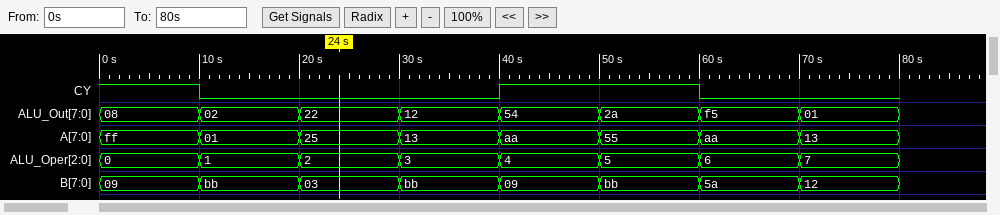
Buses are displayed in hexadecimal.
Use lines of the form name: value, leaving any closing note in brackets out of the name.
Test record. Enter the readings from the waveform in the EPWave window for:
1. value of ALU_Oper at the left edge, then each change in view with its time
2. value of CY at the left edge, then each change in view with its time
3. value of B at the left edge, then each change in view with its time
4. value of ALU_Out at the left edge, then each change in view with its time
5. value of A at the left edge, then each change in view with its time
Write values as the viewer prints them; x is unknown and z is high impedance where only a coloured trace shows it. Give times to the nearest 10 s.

value of ALU_Oper at the left edge, then each change in view with its time: 0, 1 at 10 s, 2 at 20 s, 3 at 30 s, 4 at 40 s, 5 at 50 s, 6 at 60 s, 7 at 70 s
value of CY at the left edge, then each change in view with its time: 1, 0 at 10 s, 1 at 40 s, 0 at 60 s
value of B at the left edge, then each change in view with its time: 09, bb at 10 s, 03 at 20 s, bb at 30 s, 09 at 40 s, bb at 50 s, 5a at 60 s, 12 at 70 s
value of ALU_Out at the left edge, then each change in view with its time: 08, 02 at 10 s, 22 at 20 s, 12 at 30 s, 54 at 40 s, 2a at 50 s, f5 at 60 s, 01 at 70 s
value of A at the left edge, then each change in view with its time: ff, 01 at 10 s, 25 at 20 s, 13 at 30 s, aa at 40 s, 55 at 50 s, aa at 60 s, 13 at 70 s
